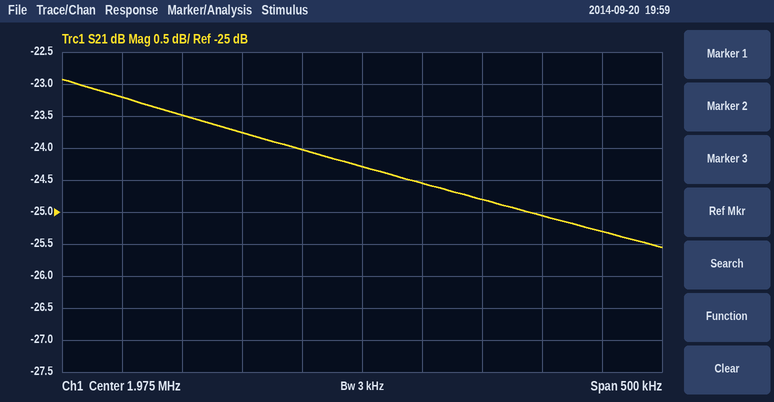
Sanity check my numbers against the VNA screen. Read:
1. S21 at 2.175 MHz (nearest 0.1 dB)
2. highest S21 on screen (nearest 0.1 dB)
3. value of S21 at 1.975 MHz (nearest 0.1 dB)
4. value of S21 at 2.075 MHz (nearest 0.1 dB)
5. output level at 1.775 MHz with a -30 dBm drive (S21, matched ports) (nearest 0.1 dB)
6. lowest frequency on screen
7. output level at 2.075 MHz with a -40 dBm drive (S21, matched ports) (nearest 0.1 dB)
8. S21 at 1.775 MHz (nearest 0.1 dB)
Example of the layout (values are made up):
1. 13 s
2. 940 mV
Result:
1. -25.3 dB
2. -22.9 dB
3. -24.3 dB
4. -24.8 dB
5. -53.2 dBm
6. 1.725 MHz
7. -64.8 dBm
8. -23.2 dB
